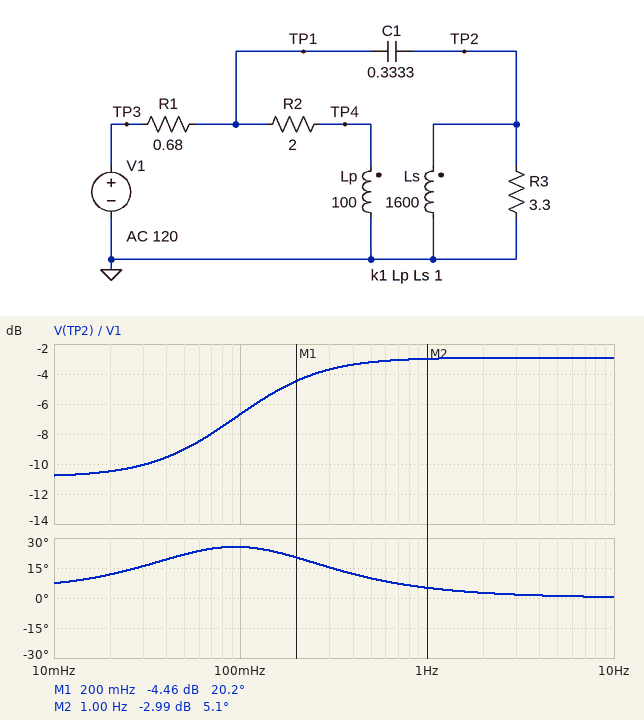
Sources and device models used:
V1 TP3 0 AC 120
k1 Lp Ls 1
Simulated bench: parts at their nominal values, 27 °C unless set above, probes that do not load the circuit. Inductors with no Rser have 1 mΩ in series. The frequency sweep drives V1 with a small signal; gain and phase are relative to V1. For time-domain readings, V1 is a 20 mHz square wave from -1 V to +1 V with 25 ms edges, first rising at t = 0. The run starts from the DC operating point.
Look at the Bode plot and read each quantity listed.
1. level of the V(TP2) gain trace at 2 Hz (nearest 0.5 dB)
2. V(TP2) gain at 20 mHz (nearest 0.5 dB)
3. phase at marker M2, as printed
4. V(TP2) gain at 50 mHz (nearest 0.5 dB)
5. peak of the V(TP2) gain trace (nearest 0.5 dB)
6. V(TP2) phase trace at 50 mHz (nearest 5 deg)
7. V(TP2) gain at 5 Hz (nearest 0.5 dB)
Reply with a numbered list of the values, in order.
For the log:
1. -3.0 dB
2. -10.5 dB
3. 5.1 deg
4. -9.0 dB
5. -3.0 dB
6. 20 deg
7. -3.0 dB
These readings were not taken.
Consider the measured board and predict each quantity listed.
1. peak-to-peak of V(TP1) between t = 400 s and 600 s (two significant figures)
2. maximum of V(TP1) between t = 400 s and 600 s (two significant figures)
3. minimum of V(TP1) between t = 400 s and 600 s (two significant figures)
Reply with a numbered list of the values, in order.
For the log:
1. 1.5 V
2. 770 mV
3. -760 mV
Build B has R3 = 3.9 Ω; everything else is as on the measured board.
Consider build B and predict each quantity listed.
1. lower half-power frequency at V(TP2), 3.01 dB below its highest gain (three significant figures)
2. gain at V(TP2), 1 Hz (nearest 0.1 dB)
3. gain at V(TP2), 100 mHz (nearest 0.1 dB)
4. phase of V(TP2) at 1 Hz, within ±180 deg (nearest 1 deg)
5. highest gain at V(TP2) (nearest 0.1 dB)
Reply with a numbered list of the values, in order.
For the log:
1. 99.9 mHz
2. -2.8 dB
3. -5.7 dB
4. 4 deg
5. -2.7 dB
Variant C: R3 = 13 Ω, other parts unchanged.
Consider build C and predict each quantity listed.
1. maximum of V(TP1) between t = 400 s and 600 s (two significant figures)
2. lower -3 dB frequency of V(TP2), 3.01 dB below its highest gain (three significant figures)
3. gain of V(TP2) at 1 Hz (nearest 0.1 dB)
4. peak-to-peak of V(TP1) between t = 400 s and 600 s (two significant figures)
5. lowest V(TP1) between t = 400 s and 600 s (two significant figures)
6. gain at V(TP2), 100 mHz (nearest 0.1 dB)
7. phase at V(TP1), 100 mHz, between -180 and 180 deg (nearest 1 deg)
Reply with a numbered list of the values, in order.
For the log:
1. 810 mV
2. 991 µHz
3. -1.9 dB
4. 1.6 V
5. -810 mV
6. -1.6 dB
7. 0 deg
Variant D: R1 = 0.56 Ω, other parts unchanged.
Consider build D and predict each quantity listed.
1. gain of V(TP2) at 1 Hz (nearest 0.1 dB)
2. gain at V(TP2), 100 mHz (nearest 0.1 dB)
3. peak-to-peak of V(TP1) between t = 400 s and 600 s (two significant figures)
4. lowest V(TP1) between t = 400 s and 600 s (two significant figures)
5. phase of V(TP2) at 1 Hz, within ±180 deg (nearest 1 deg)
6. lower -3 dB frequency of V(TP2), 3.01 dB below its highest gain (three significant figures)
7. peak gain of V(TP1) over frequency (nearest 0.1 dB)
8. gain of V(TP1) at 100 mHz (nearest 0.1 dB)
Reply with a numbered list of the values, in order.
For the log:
1. -2.5 dB
2. -6.3 dB
3. 1.6 V
4. -790 mV
5. 5 deg
6. 125 mHz
7. -2.0 dB
8. -2.1 dB
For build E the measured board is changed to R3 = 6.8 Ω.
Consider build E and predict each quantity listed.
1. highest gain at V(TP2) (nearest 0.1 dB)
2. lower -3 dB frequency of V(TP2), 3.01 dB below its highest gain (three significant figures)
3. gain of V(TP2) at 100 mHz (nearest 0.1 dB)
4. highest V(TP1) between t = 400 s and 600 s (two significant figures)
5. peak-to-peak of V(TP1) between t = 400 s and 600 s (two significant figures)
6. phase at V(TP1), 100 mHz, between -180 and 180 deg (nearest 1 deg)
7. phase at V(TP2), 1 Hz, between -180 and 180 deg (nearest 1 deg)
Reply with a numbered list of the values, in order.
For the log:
1. -2.2 dB
2. 4.83 mHz
3. -3.2 dB
4. 790 mV
5. 1.6 V
6. 0 deg
7. 1 deg
